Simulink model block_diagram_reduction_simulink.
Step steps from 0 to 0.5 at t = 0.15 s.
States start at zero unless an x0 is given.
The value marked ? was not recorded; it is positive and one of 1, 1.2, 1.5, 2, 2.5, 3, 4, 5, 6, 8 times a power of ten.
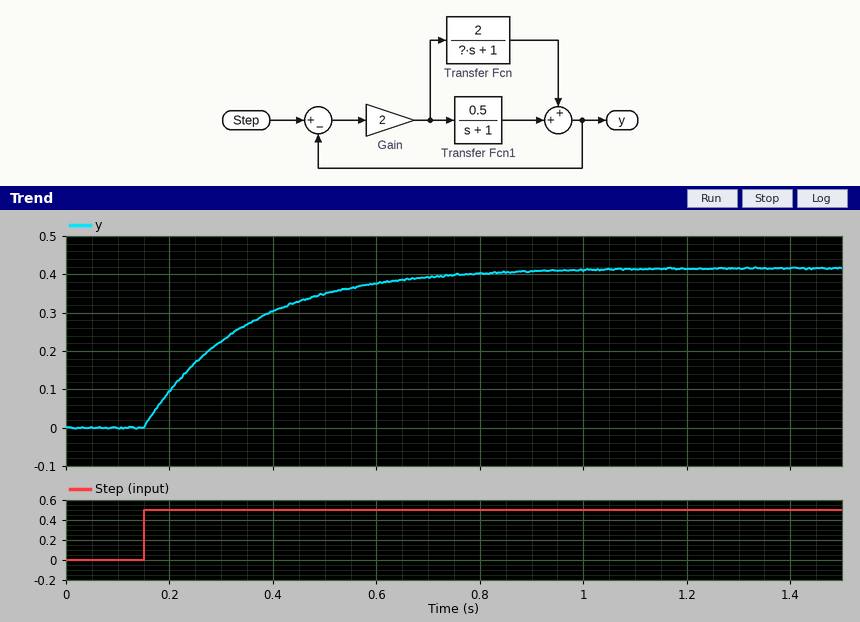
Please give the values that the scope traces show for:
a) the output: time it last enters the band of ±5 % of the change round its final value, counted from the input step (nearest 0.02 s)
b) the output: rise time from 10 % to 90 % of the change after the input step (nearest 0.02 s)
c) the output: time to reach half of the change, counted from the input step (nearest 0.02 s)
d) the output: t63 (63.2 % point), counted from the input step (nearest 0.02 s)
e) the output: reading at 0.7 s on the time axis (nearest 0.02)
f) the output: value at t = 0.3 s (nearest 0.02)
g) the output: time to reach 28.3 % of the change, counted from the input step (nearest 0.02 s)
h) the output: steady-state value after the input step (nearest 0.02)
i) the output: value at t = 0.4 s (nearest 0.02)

0.58 s
0.42 s
0.14 s
0.20 s
0.40
0.22
0.06 s
0.42
0.30
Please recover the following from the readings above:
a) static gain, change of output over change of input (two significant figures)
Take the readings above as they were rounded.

0.84
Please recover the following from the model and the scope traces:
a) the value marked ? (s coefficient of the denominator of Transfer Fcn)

1.2
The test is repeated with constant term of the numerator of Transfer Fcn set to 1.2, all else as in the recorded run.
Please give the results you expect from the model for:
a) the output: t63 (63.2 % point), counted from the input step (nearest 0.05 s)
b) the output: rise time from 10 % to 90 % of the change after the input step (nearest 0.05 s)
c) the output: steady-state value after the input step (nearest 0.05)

0.25 s
0.55 s
0.40
